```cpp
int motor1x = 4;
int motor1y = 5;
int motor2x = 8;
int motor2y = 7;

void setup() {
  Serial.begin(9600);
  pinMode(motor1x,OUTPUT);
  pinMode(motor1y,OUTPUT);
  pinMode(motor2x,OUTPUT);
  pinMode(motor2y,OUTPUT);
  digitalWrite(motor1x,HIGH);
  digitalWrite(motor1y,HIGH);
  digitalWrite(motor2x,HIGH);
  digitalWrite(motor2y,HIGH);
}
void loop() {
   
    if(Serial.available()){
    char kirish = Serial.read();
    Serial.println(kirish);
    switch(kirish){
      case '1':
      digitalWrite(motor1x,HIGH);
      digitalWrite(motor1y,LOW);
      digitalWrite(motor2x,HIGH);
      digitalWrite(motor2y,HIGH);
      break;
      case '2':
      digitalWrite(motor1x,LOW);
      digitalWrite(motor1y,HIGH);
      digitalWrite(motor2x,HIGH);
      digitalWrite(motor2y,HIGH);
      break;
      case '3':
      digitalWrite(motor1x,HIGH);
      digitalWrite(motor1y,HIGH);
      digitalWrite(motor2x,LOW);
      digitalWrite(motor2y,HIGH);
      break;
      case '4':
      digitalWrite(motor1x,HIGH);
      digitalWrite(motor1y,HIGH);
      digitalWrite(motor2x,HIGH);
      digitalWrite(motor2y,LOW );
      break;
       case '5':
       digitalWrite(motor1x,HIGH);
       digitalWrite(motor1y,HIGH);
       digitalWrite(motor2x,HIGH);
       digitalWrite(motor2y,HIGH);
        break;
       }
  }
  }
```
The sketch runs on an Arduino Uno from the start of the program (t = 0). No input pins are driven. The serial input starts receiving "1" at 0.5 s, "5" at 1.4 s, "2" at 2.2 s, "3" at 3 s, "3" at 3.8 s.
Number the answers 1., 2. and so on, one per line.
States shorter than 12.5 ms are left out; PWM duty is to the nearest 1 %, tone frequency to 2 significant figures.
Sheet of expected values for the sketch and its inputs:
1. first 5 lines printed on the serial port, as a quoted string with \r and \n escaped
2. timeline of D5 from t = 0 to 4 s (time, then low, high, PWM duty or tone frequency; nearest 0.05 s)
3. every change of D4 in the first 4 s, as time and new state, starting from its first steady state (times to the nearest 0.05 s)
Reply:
1. "1\r\n5\r\n2\r\n3\r\n3\r\n"
2. 0 s high; 0.5 s low; 1.4 s high
3. 0 s high; 2.2 s low; 3 s high
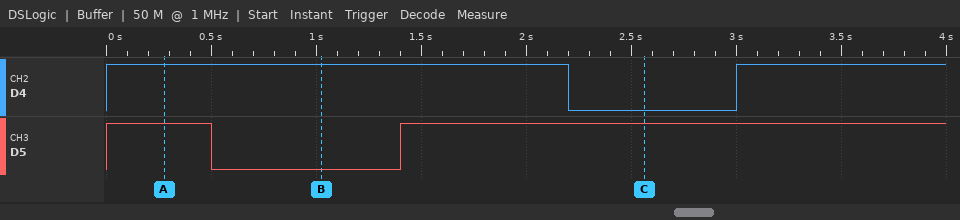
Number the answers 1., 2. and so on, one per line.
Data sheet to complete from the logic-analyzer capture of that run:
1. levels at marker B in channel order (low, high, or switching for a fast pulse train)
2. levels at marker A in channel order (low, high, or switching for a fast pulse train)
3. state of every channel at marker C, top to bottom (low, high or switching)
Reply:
1. D4 high, D5 low
2. D4 high, D5 high
3. D4 low, D5 high
